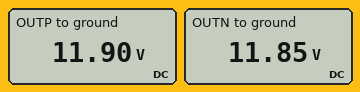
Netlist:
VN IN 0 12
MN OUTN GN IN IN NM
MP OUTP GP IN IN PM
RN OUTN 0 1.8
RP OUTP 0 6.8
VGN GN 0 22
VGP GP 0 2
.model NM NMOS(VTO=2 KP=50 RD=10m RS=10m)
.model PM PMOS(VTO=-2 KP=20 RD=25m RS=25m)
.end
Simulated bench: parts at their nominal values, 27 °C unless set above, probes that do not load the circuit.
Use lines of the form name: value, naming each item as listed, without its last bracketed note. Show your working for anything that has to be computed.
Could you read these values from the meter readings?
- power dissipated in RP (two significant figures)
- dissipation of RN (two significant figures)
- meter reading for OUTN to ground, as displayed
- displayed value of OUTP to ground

power dissipated in RP: (11.9 V)^2 / 6.8 Ω = 21 W
dissipation of RN: (11.85 V)^2 / 1.8 Ω = 78 W
meter reading for OUTN to ground, as displayed: 11.85 V
displayed value of OUTP to ground: 11.90 V
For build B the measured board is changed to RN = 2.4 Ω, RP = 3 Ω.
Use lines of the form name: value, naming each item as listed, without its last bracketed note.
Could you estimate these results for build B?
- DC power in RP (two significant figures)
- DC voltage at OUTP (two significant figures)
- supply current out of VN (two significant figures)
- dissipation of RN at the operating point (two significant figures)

DC power in RP: 46 W
DC voltage at OUTP: 12 V
supply current out of VN: 8.9 A
dissipation of RN at the operating point: 59 W
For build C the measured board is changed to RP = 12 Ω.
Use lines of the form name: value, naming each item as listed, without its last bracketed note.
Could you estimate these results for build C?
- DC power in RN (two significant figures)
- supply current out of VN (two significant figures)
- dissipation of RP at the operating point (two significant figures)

DC power in RN: 78 W
supply current out of VN: 7.6 A
dissipation of RP at the operating point: 12 W
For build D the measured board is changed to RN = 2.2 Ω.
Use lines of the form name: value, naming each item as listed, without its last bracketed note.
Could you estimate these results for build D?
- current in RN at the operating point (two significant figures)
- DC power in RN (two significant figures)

current in RN at the operating point: 5.4 A
DC power in RN: 64 W
